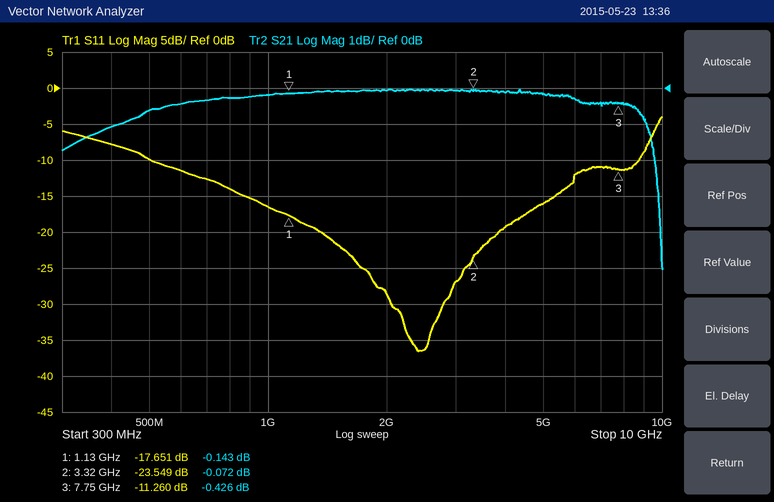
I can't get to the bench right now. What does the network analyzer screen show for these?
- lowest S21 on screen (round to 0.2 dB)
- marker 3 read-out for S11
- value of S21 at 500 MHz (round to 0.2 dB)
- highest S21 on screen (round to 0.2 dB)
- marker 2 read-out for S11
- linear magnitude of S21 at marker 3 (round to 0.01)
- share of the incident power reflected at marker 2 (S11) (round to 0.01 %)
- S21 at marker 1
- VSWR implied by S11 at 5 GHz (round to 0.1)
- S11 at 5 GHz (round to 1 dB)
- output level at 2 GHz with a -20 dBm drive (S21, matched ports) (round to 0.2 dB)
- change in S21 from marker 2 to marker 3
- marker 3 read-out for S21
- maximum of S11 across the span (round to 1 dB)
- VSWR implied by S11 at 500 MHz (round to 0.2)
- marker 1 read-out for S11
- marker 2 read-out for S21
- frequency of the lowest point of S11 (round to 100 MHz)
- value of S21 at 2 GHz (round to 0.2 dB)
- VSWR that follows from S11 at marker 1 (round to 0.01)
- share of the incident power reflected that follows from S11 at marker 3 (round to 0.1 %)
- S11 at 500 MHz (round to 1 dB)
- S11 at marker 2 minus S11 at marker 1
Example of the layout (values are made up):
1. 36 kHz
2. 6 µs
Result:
1. -5.0 dB
2. -11.260 dB
3. -0.6 dB
4. 0.0 dB
5. -23.549 dB
6. 0.95
7. 0.44 %
8. -0.143 dB
9. 1.4
10. -16 dB
11. -20.0 dBm
12. -0.354 dB
13. -0.426 dB
14. -4 dB
15. 2.0
16. -17.651 dB
17. -0.072 dB
18. 2.4 GHz
19. 0.0 dB
20. 1.30
21. 7.5 %
22. -10 dB
23. -5.898 dB
